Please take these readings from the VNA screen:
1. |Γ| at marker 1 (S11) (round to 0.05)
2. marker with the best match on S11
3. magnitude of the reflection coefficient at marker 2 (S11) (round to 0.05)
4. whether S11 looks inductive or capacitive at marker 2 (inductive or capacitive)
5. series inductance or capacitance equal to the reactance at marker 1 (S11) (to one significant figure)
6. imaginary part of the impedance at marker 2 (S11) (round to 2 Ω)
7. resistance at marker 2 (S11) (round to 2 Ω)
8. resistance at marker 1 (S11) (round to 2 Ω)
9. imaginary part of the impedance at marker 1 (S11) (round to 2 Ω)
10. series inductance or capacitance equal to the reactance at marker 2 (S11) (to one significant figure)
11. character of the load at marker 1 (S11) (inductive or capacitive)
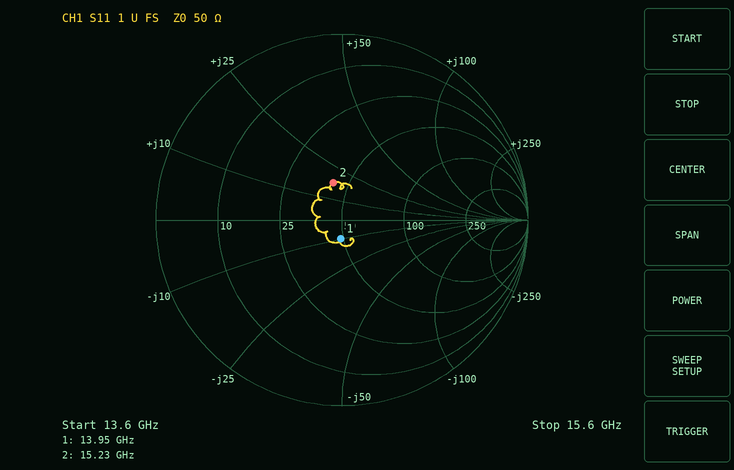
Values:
0.10
marker 1
0.20
inductive
1 pF
+18 Ω
42 Ω
48 Ω
-10 Ω
200 pH
capacitive
